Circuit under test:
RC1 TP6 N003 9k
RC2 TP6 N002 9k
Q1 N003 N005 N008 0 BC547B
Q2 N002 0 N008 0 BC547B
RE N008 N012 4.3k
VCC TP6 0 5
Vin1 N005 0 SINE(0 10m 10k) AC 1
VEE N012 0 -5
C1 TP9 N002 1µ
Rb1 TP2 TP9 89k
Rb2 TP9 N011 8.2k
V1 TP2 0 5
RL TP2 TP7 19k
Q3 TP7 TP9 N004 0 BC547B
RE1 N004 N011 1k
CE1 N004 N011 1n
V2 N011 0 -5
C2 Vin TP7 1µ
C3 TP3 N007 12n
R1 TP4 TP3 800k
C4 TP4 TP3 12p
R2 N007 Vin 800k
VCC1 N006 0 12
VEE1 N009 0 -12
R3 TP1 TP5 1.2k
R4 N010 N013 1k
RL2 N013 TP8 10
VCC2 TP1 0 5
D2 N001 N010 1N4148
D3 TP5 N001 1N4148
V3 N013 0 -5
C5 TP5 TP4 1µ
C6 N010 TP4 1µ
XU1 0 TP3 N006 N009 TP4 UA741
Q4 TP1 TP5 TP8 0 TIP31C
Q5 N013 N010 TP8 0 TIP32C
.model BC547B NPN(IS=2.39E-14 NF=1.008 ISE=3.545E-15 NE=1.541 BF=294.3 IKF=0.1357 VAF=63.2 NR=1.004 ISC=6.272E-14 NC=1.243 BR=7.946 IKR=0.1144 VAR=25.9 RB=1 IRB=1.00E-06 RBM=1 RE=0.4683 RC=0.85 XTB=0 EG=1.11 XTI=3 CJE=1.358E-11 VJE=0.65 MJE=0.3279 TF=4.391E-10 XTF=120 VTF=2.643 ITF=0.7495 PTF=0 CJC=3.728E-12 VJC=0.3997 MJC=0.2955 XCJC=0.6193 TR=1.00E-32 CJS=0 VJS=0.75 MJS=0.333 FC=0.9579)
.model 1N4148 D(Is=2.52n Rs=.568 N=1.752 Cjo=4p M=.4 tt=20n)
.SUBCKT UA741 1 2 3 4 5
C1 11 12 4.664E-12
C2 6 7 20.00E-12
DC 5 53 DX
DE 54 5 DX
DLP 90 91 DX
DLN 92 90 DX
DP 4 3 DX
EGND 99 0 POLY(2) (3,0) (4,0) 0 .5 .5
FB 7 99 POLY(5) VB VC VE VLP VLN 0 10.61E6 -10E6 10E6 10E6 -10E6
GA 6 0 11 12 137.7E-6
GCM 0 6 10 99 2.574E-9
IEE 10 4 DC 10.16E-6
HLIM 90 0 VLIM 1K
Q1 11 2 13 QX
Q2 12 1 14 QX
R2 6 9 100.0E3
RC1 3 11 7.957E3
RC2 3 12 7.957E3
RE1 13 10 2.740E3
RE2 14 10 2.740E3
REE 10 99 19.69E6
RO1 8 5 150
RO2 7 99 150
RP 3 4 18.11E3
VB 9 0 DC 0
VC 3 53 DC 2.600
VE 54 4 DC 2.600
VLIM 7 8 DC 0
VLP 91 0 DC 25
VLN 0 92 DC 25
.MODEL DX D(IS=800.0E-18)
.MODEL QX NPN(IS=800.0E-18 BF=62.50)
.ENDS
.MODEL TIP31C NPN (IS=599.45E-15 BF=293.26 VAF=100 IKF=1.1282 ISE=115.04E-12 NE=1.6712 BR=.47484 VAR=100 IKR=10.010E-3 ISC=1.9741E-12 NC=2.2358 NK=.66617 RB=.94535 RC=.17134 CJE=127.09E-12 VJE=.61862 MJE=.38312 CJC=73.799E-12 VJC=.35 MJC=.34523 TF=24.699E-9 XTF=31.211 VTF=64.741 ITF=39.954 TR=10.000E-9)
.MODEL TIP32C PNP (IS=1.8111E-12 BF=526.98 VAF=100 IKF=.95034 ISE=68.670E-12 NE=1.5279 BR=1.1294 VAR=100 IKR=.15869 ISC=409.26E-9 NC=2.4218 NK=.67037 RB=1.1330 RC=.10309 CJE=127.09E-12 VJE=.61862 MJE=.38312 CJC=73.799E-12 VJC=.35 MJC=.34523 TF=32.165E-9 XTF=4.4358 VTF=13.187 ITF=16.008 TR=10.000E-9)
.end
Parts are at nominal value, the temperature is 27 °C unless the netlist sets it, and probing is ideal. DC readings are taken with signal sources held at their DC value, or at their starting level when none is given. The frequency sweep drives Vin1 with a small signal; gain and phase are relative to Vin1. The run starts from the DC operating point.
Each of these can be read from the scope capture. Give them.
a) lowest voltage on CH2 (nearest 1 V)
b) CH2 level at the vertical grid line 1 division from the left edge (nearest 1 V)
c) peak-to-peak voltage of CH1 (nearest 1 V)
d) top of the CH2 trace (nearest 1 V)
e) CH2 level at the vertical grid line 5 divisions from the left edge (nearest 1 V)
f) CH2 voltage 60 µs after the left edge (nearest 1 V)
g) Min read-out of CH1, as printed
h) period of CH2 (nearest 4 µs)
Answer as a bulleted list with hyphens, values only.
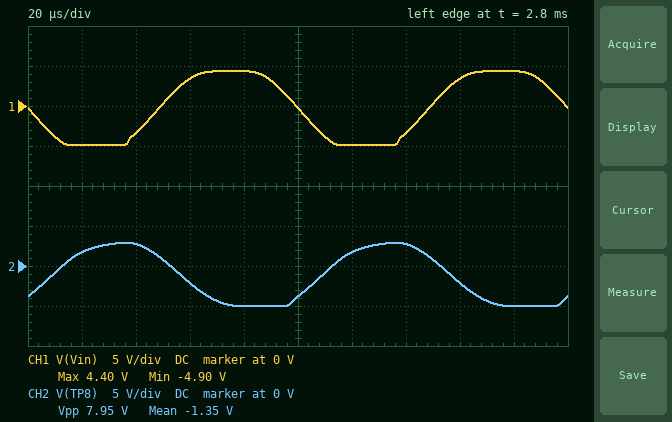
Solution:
- -5 V
- 2 V
- 9 V
- 3 V
- -4 V
- -2 V
- -4.90 V
- 100 µs
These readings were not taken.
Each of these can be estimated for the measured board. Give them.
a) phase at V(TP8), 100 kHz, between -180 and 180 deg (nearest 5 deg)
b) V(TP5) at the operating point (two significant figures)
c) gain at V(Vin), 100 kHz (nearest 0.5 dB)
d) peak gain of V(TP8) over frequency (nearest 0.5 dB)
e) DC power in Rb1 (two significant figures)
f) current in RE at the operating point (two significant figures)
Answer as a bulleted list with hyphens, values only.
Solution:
- -70 deg
- -1.2 V
- 57.5 dB
- 55.5 dB
- 940 µW
- 1.0 mA
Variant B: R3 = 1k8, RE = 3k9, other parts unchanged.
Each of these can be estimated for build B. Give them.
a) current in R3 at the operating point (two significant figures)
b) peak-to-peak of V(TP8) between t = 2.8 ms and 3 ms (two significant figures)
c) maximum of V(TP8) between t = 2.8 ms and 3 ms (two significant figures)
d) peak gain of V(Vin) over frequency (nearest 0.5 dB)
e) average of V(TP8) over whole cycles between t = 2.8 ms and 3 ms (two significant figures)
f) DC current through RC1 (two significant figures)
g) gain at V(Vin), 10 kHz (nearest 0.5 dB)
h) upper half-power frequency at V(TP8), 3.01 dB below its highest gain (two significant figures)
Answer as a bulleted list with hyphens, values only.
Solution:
- 3.9 mA
- 7.2 V
- 2.2 V
- 67.5 dB
- -1.8 V
- 560 µA
- 56.5 dB
- 17 kHz
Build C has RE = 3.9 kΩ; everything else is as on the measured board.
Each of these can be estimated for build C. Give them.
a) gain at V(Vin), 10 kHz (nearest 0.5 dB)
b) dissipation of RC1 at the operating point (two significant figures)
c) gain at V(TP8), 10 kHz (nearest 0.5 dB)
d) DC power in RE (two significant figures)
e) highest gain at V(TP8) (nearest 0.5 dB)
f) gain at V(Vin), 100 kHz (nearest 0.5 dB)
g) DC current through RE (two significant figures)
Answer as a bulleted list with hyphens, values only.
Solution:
- 56.5 dB
- 2.8 mW
- 55.0 dB
- 4.9 mW
- 56.0 dB
- 58.0 dB
- 1.1 mA
